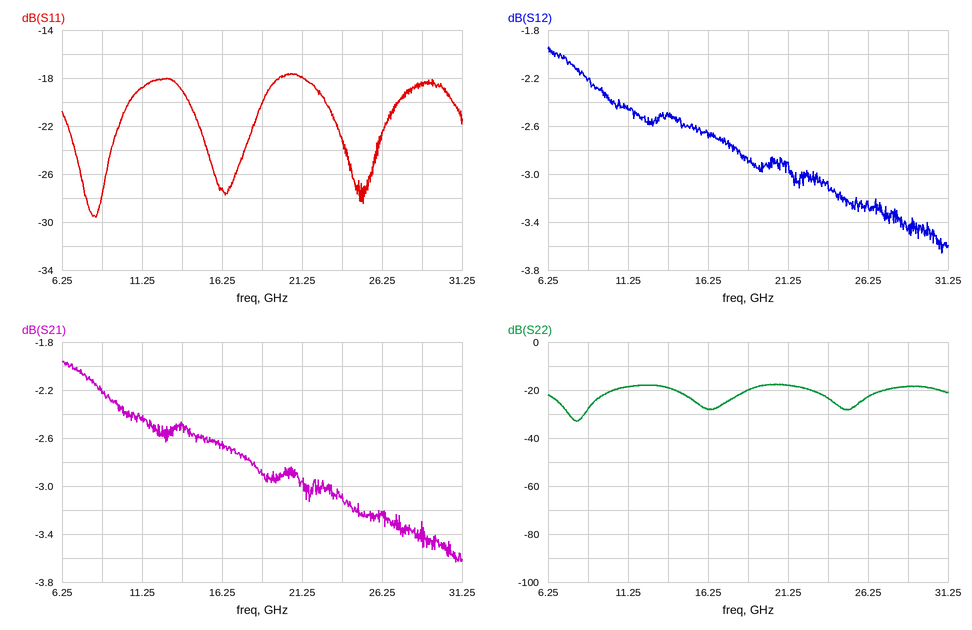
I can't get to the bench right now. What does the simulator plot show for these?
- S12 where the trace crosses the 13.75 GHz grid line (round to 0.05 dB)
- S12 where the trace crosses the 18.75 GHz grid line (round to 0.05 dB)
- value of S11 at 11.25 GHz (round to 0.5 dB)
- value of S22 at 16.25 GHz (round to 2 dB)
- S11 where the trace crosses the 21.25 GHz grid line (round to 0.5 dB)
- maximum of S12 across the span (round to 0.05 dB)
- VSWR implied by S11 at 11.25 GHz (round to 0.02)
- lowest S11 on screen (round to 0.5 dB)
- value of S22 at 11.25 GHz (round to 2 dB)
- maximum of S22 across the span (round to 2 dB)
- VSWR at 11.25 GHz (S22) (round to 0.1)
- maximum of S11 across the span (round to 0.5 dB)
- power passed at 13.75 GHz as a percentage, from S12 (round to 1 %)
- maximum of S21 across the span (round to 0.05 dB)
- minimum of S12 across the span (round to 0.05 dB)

-2.50 dB
-2.90 dB
-19.0 dB
-28 dB
-18.0 dB
-1.95 dB
1.26
-29.5 dB
-18 dB
-18 dB
1.3
-17.5 dB
56 %
-1.95 dB
-3.65 dB
